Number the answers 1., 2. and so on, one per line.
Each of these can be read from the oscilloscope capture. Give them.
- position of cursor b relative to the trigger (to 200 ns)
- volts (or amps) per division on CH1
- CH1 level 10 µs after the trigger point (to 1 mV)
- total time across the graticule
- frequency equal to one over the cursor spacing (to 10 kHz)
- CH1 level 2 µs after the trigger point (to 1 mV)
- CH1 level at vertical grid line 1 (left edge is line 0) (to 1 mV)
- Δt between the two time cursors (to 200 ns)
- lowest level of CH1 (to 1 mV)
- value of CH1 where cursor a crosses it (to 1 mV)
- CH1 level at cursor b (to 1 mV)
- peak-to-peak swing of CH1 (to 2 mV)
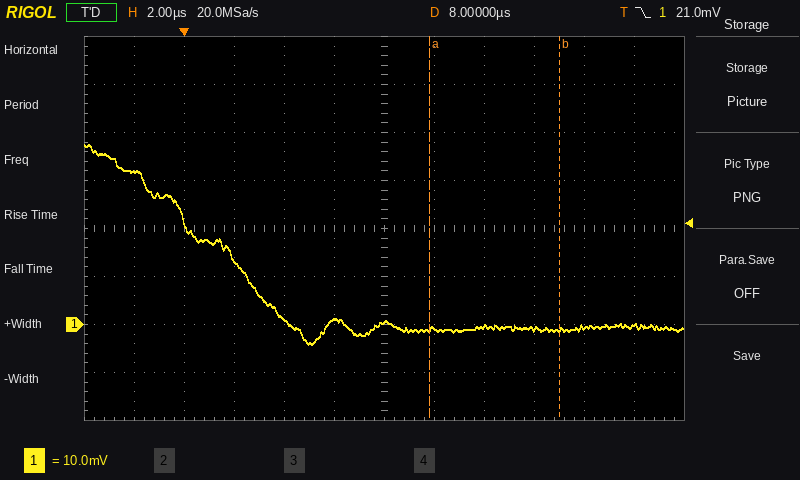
1. +15.0 µs
2. 10 mV
3. -1 mV
4. 24 µs
5. 190 kHz
6. 14 mV
7. 32 mV
8. 5.2 µs
9. -4 mV
10. -1 mV
11. -1 mV
12. 42 mV
